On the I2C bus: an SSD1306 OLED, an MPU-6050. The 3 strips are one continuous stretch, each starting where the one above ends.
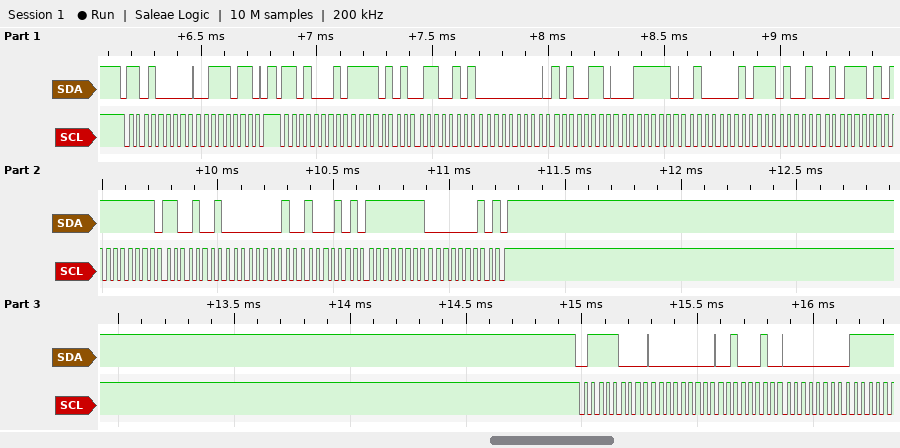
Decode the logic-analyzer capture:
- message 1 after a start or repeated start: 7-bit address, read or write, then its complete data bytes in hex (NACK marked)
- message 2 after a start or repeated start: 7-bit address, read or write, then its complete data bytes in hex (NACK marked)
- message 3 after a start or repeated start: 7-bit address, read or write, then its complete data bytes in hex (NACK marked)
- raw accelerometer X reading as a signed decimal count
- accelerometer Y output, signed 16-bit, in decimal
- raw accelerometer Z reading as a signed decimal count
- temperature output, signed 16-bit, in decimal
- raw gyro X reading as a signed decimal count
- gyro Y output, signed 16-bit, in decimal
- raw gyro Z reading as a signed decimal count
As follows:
0x68 write: 3B
0x68 read: F5 65 00 A6 3E 41 E9 5D FF C9 01 45 FF 02 NACK
0x3C write: 00 22 00
-2715
166
15937
-5795
-55
325
-254
